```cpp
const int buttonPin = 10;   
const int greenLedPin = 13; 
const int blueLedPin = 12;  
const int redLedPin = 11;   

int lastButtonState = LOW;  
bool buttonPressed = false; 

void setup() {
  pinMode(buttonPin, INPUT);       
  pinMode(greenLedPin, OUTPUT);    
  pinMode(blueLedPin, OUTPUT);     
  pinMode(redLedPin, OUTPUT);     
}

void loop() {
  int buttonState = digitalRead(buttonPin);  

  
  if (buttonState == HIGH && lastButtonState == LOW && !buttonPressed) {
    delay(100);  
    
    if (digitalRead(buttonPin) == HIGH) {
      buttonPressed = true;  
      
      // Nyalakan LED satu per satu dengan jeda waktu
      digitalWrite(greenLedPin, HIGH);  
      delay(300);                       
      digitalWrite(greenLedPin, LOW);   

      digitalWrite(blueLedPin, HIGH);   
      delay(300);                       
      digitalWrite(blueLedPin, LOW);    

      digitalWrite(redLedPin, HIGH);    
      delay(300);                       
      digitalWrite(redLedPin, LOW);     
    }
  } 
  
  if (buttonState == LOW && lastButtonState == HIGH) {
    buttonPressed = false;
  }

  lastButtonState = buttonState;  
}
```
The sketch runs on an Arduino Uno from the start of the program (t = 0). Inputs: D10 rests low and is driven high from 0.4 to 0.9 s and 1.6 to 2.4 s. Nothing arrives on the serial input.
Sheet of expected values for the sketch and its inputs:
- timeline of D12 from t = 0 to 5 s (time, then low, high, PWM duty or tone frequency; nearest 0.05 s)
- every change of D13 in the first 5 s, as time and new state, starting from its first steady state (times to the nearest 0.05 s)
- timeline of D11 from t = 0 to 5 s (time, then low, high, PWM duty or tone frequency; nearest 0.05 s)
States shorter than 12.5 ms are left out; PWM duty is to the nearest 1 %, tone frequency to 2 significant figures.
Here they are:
0 s low; 0.8 s high; 1.1 s low; 2 s high; 2.3 s low
0 s low; 0.5 s high; 0.8 s low; 1.7 s high; 2 s low
0 s low; 1.1 s high; 1.4 s low; 2.3 s high; 2.6 s low
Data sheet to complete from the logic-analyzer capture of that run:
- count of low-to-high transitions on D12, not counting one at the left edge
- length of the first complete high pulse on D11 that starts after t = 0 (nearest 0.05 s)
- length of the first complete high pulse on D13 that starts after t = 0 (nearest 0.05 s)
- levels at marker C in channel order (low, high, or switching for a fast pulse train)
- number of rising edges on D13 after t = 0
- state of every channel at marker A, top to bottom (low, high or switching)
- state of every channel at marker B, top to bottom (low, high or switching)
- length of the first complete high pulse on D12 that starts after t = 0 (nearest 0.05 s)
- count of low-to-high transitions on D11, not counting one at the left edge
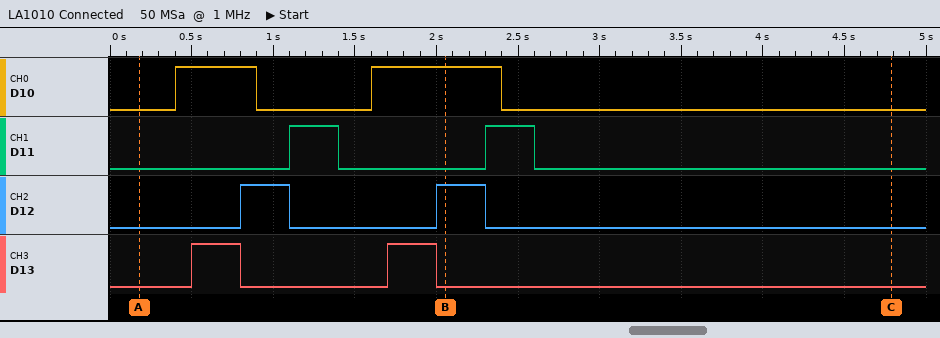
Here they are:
2
0.30 s
0.30 s
D10 low, D11 low, D12 low, D13 low
2
D10 low, D11 low, D12 low, D13 low
D10 high, D11 low, D12 high, D13 low
0.30 s
2
